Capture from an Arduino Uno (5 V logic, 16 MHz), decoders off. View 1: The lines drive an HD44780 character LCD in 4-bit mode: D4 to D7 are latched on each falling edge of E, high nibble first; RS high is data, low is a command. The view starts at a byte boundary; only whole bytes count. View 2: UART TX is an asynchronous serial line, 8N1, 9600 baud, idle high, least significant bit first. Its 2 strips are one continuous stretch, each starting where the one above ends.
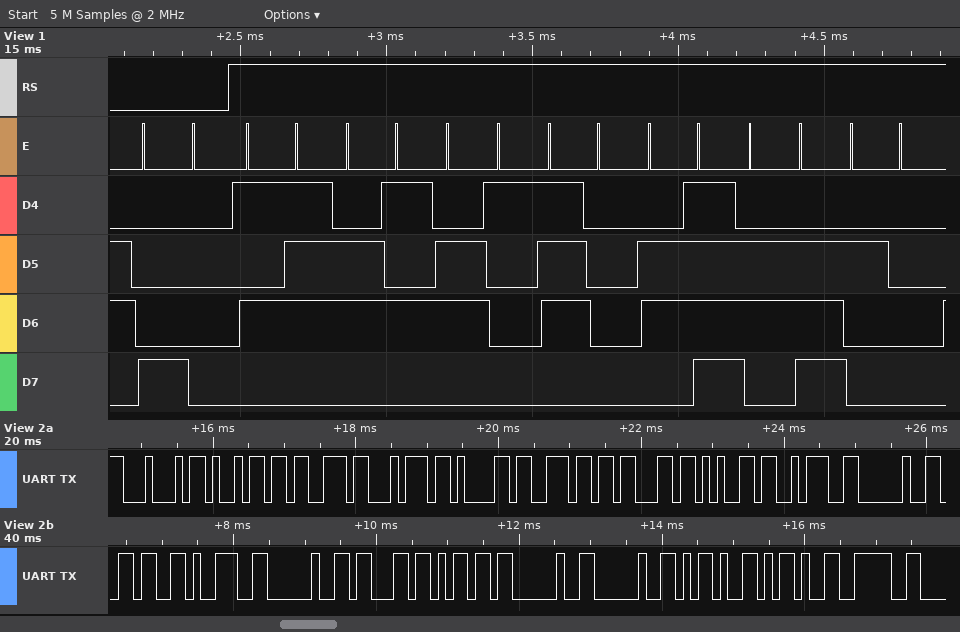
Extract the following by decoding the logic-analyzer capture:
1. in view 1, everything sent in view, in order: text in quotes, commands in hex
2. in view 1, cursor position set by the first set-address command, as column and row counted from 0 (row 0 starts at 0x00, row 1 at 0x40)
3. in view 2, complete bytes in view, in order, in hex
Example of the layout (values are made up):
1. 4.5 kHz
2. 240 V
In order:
1. 0x80 "Weapon "
2. column 0, row 0
3. 44 69 73 74 61 6E 63 65 3A 20 36 39 20 63 6D 20 20 2D 2D 3E
